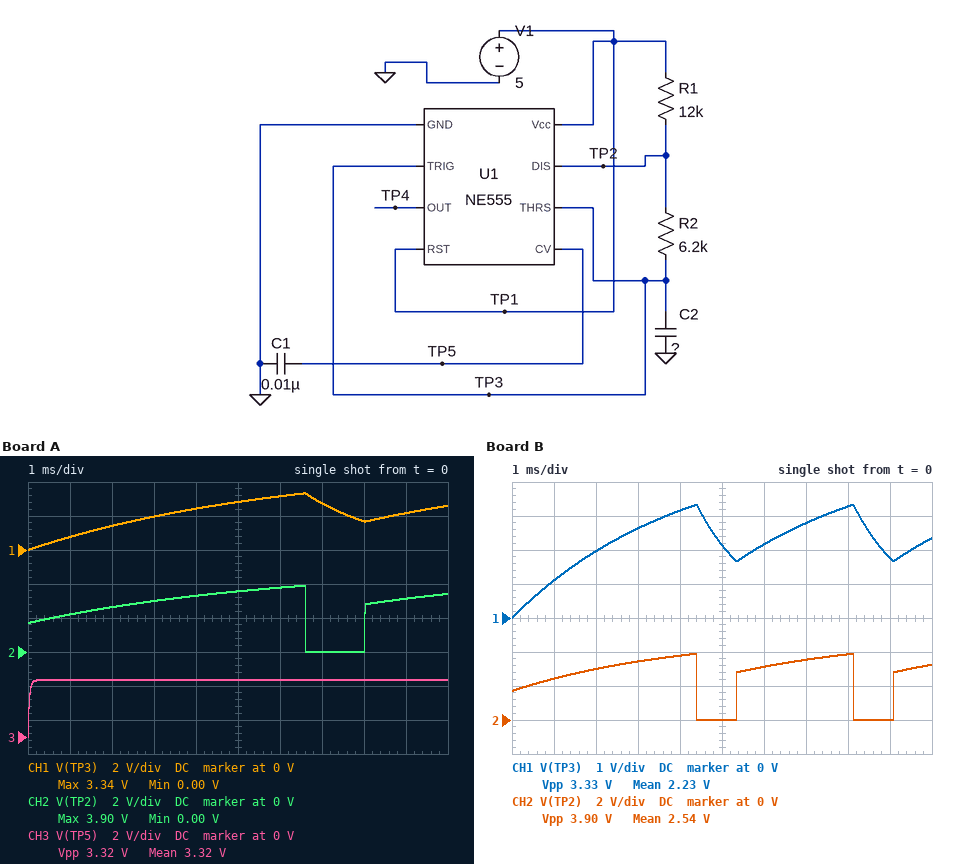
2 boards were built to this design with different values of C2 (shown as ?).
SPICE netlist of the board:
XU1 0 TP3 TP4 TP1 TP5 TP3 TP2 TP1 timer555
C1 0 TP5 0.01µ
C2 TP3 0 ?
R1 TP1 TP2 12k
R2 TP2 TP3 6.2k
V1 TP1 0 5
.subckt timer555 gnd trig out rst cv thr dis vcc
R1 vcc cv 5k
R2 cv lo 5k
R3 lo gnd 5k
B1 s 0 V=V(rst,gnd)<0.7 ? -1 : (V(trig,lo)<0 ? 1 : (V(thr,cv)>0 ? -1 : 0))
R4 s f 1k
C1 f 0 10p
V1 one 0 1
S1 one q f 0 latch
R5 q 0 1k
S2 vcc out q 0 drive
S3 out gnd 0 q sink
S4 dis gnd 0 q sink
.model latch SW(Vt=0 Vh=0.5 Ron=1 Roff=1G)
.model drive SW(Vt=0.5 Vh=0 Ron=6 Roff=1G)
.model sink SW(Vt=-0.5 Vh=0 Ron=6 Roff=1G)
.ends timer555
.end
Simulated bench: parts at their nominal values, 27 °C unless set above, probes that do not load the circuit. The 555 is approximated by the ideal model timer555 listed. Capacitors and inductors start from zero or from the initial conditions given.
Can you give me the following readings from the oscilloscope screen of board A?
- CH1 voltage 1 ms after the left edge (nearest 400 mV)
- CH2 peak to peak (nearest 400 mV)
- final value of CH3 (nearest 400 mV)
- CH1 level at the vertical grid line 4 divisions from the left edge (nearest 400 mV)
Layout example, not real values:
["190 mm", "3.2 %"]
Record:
["800 mV", "4.0 V", "3.2 V", "2.4 V"]
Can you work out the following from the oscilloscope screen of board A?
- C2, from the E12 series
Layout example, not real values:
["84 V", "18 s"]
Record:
["330 nF"]
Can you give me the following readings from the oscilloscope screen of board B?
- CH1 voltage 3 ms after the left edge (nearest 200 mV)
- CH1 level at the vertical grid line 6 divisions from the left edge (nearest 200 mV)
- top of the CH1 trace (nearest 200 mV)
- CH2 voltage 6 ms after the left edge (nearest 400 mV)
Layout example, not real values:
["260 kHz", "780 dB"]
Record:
["2.6 V", "2.2 V", "3.4 V", "3.2 V"]
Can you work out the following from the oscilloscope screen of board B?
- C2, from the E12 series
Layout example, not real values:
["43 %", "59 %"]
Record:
["220 nF"]
